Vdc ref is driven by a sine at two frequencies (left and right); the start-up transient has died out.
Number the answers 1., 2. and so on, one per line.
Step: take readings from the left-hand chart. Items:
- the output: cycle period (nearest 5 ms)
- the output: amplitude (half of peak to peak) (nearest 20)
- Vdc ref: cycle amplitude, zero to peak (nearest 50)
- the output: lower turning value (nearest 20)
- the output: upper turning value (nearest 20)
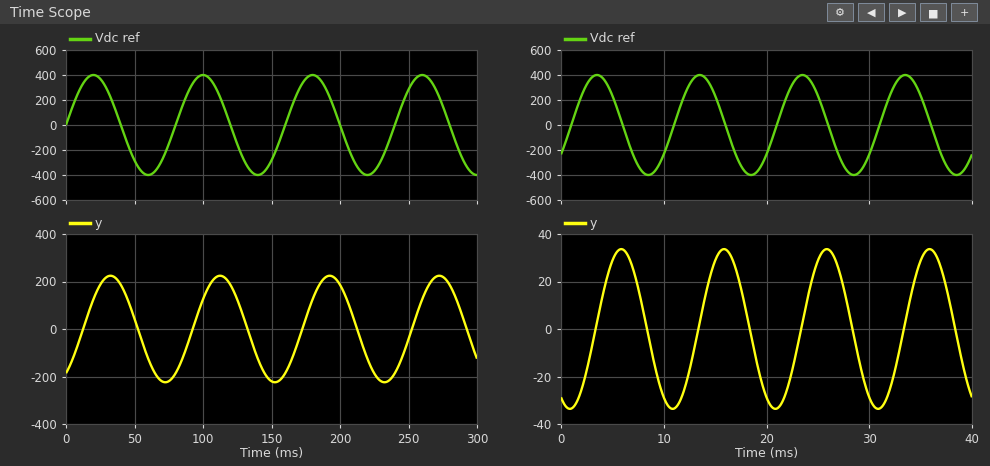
1. 80 ms
2. 220
3. 400
4. -220
5. 220
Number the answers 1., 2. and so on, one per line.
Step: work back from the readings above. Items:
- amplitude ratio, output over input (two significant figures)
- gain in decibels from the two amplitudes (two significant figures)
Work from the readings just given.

1. 0.55
2. -5.2 dB
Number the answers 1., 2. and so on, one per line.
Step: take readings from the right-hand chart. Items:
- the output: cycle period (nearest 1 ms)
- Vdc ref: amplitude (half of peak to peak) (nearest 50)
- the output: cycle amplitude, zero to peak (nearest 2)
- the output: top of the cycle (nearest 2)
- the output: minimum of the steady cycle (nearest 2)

1. 10 ms
2. 400
3. 34
4. 34
5. -34
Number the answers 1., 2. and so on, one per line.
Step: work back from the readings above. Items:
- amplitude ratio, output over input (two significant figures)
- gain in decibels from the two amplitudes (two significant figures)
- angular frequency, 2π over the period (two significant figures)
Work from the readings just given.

1. 0.085
2. -21 dB
3. 0.63 rad/ms
